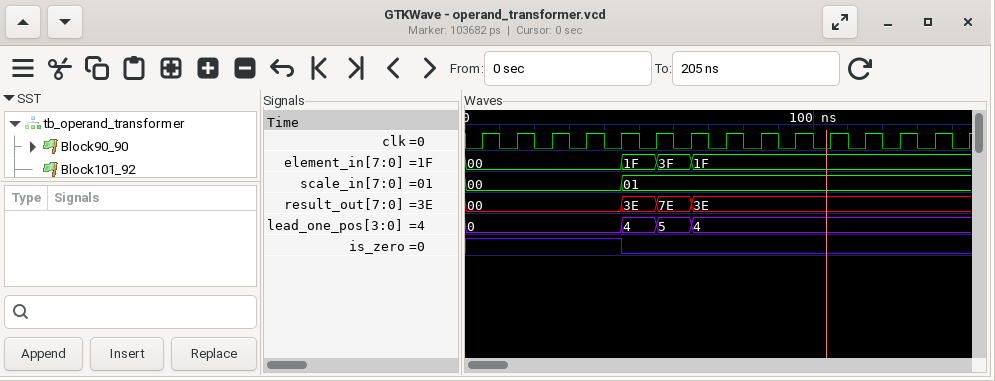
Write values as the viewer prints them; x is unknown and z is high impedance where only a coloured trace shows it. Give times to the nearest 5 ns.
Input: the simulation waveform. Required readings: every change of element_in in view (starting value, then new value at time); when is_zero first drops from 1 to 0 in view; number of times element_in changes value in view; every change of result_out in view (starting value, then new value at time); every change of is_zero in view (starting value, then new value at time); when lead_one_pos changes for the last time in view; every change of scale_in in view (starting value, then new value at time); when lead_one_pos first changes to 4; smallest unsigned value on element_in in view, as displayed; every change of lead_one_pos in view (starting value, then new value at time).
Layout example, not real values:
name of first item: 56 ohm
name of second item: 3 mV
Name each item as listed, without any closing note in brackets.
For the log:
every change of element_in in view: 00, 1F at 45 ns, 3F at 55 ns, 1F at 65 ns
when is_zero first drops from 1 to 0 in view: 45 ns
number of times element_in changes value in view: 3
every change of result_out in view: 00, 3E at 45 ns, 7E at 55 ns, 3E at 65 ns
every change of is_zero in view: 1, 0 at 45 ns
when lead_one_pos changes for the last time in view: 65 ns
every change of scale_in in view: 00, 01 at 45 ns
when lead_one_pos first changes to 4: 45 ns
smallest unsigned value on element_in in view, as displayed: 00
every change of lead_one_pos in view: 0, 4 at 45 ns, 5 at 55 ns, 4 at 65 ns
